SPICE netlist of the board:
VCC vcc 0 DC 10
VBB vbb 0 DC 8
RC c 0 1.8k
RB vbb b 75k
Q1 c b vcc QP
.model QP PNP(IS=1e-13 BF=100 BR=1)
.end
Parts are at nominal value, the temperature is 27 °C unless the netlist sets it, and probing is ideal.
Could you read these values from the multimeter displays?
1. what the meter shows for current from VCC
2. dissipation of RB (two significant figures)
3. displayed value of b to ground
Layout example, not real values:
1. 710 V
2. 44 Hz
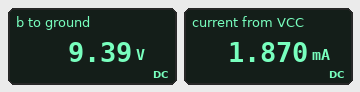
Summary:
1. 1.870 mA
2. 26 µW
3. 9.39 V
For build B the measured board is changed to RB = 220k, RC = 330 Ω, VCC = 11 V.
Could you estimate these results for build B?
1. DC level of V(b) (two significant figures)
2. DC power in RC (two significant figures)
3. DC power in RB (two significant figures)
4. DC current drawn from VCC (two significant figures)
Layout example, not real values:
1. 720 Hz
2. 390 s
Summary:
1. 10 V
2. 390 µW
3. 26 µW
4. 1.1 mA
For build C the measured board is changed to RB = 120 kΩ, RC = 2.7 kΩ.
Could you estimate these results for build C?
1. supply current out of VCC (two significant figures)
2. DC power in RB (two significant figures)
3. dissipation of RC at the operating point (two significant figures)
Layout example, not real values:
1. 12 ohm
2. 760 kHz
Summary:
1. 1.2 mA
2. 16 µW
3. 3.7 mW
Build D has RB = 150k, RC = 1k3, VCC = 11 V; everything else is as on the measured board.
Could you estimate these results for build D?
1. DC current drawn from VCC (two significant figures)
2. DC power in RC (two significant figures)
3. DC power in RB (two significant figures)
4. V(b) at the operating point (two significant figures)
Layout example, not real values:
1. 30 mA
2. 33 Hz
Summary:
1. 1.6 mA
2. 3.3 mW
3. 38 µW
4. 10 V
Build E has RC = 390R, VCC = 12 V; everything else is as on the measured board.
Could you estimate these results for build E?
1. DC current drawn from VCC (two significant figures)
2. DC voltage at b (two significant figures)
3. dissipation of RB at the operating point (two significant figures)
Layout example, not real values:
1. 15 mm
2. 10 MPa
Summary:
1. 4.5 mA
2. 11 V
3. 150 µW
